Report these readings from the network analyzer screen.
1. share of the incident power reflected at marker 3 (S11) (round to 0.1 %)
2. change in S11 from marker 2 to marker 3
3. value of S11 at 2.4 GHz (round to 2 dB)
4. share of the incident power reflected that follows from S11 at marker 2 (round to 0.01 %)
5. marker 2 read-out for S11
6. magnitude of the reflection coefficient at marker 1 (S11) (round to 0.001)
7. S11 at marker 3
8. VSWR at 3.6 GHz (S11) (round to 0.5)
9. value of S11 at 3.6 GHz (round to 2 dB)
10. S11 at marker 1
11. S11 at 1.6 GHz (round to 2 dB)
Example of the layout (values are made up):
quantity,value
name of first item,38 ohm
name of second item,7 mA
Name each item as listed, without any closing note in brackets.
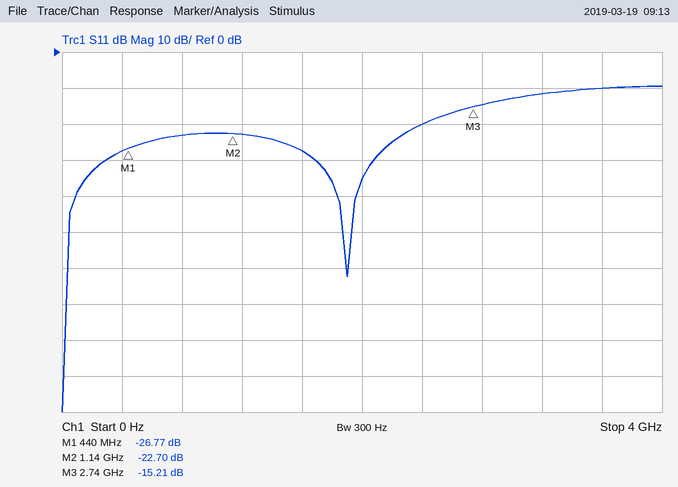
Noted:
quantity,value
share of the incident power reflected at marker 3 (S11),3.0 %
change in S11 from marker 2 to marker 3,7.49 dB
value of S11 at 2.4 GHz,-20 dB
share of the incident power reflected that follows from S11 at marker 2,0.54 %
marker 2 read-out for S11,-22.70 dB
magnitude of the reflection coefficient at marker 1 (S11),0.046
S11 at marker 3,-15.21 dB
VSWR at 3.6 GHz (S11),2.0
value of S11 at 3.6 GHz,-10 dB
S11 at marker 1,-26.77 dB
S11 at 1.6 GHz,-28 dB
